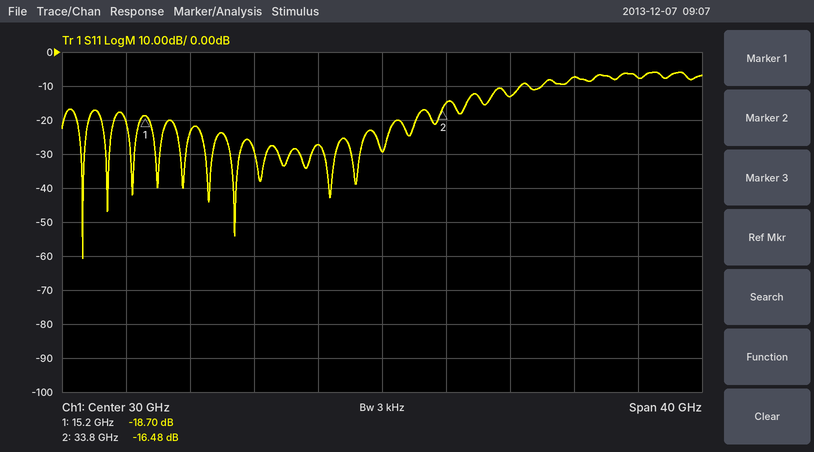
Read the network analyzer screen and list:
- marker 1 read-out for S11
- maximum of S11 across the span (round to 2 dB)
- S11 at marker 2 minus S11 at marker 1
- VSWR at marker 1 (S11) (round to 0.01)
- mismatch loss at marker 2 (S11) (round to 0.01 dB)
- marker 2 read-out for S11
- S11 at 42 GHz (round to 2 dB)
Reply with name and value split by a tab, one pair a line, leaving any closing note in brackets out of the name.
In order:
marker 1 read-out for S11	-18.70 dB
maximum of S11 across the span	-6 dB
S11 at marker 2 minus S11 at marker 1	2.22 dB
VSWR at marker 1 (S11)	1.26
mismatch loss at marker 2 (S11)	0.10 dB
marker 2 read-out for S11	-16.48 dB
S11 at 42 GHz	-8 dB
